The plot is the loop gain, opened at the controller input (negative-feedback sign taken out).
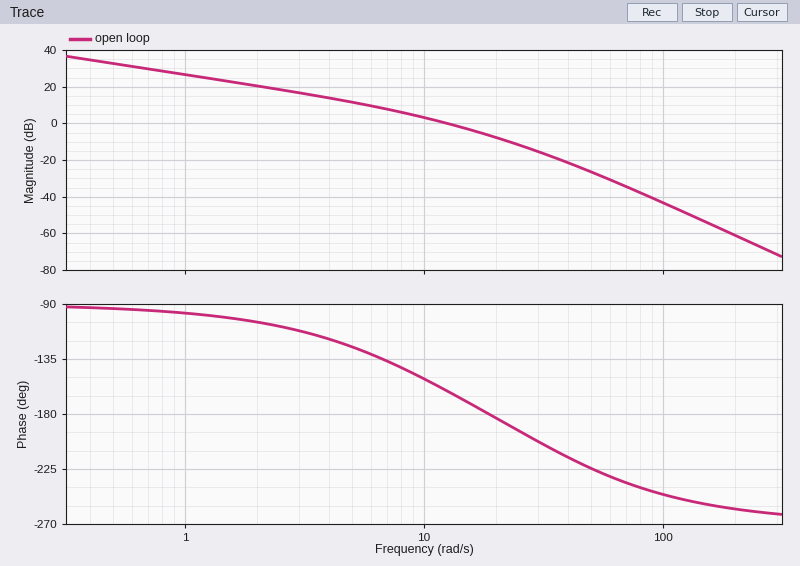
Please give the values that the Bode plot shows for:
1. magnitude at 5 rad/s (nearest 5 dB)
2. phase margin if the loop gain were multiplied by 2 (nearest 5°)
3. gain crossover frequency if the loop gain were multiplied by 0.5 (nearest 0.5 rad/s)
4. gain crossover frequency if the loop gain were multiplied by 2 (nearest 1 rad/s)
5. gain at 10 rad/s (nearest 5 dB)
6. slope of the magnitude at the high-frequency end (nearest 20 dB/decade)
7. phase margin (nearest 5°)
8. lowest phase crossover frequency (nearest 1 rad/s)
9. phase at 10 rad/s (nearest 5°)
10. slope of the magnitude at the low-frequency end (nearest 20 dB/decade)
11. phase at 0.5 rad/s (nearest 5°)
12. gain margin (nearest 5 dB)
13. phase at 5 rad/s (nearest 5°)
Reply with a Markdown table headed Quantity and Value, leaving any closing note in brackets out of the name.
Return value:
| Quantity | Value |
|---|---|
| magnitude at 5 rad/s | 10 dB |
| phase margin if the loop gain were multiplied by 2 | 0° |
| gain crossover frequency if the loop gain were multiplied by 0.5 | 8.0 rad/s |
| gain crossover frequency if the loop gain were multiplied by 2 | 18 rad/s |
| gain at 10 rad/s | 5 dB |
| slope of the magnitude at the high-frequency end | -60 dB/decade |
| phase margin | 20° |
| lowest phase crossover frequency | 19 rad/s |
| phase at 10 rad/s | -150° |
| slope of the magnitude at the low-frequency end | -20 dB/decade |
| phase at 0.5 rad/s | -95° |
| gain margin | 5 dB |
| phase at 5 rad/s | -125° |
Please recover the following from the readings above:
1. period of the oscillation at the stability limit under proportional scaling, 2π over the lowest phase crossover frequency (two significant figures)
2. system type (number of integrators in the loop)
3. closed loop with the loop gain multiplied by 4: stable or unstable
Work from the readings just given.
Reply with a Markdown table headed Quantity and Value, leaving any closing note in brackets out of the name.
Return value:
| Quantity | Value |
|---|---|
| period of the oscillation at the stability limit under proportional scaling, 2π over the lowest phase crossover frequency | 0.33 s |
| system type | 1 |
| closed loop with the loop gain multiplied by 4: stable or unstable | unstable |
